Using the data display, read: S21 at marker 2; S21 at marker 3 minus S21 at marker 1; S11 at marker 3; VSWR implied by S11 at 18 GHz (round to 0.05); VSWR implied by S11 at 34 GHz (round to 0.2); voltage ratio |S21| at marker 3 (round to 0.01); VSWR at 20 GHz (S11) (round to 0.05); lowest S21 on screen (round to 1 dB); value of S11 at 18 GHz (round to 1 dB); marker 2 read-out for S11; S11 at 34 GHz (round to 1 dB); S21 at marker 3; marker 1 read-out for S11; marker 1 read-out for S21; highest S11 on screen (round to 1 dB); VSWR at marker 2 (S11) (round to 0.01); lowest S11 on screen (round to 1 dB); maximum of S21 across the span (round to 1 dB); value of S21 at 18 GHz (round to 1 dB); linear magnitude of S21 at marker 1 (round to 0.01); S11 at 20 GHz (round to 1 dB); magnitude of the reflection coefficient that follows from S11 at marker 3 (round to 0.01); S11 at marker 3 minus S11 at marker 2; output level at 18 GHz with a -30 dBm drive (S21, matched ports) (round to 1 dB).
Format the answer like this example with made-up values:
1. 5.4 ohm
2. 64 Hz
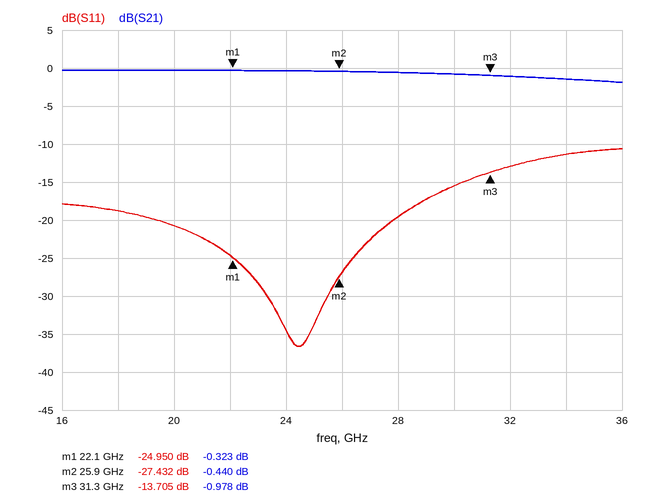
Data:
1. -0.440 dB
2. -0.655 dB
3. -13.705 dB
4. 1.25
5. 1.8
6. 0.89
7. 1.20
8. -2 dB
9. -19 dB
10. -27.432 dB
11. -11 dB
12. -0.978 dB
13. -24.950 dB
14. -0.323 dB
15. -11 dB
16. 1.09
17. -37 dB
18. 0 dB
19. 0 dB
20. 0.96
21. -21 dB
22. 0.21
23. 13.727 dB
24. -30 dBm
